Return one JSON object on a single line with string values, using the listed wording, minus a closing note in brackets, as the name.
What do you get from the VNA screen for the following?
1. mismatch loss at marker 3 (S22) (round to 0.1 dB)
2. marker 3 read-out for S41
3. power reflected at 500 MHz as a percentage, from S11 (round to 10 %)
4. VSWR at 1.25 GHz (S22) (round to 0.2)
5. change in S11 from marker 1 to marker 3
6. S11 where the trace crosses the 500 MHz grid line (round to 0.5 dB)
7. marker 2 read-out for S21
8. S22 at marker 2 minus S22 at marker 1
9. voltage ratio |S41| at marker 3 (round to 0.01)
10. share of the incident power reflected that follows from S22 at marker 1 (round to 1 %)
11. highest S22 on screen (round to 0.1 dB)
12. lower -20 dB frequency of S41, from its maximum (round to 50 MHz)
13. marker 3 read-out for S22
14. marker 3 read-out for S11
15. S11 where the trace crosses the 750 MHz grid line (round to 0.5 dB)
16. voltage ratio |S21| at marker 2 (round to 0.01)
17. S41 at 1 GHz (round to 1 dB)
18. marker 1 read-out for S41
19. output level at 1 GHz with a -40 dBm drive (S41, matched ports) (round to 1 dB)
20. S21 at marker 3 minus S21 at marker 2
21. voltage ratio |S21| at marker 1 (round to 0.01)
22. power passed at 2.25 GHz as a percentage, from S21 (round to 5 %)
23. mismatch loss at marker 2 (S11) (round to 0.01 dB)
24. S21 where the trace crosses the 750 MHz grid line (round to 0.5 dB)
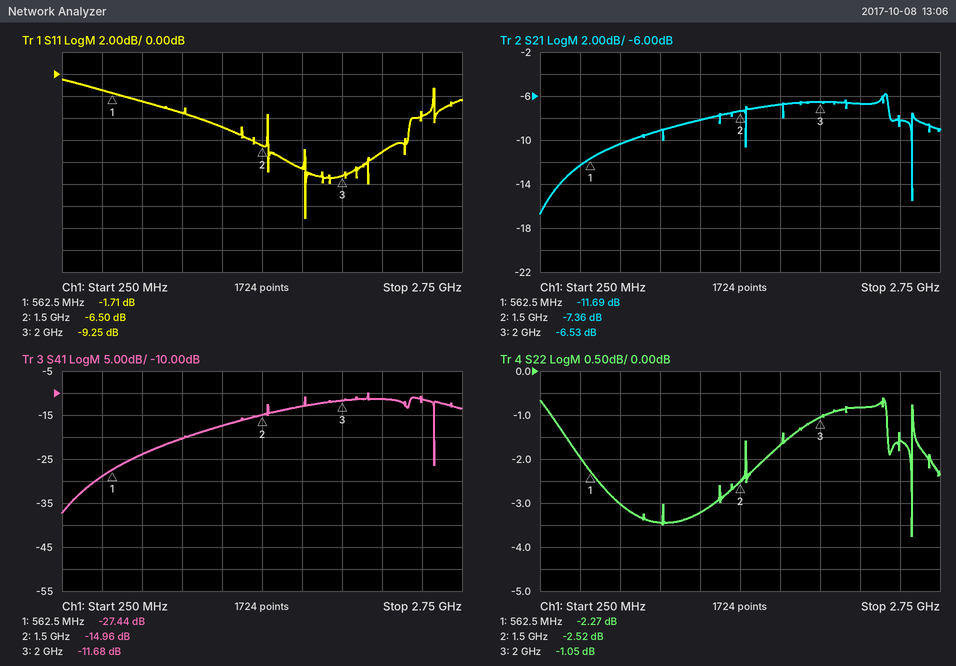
{"mismatch loss at marker 3 (S22)": "6.7 dB", "marker 3 read-out for S41": "-11.68 dB", "power reflected at 500 MHz as a percentage, from S11": "70 %", "VSWR at 1.25 GHz (S22)": "5.4", "change in S11 from marker 1 to marker 3": "-7.54 dB", "S11 where the trace crosses the 500 MHz grid line": "-1.5 dB", "marker 2 read-out for S21": "-7.36 dB", "S22 at marker 2 minus S22 at marker 1": "-0.25 dB", "voltage ratio |S41| at marker 3": "0.26", "share of the incident power reflected that follows from S22 at marker 1": "59 %", "highest S22 on screen": "-0.6 dB", "lower -20 dB frequency of S41, from its maximum": "450 MHz", "marker 3 read-out for S22": "-1.05 dB", "marker 3 read-out for S11": "-9.25 dB", "S11 where the trace crosses the 750 MHz grid line": "-2.5 dB", "voltage ratio |S21| at marker 2": "0.43", "S41 at 1 GHz": "-20 dB", "marker 1 read-out for S41": "-27.44 dB", "output level at 1 GHz with a -40 dBm drive (S41, matched ports)": "-60 dBm", "S21 at marker 3 minus S21 at marker 2": "0.83 dB", "voltage ratio |S21| at marker 1": "0.26", "power passed at 2.25 GHz as a percentage, from S21": "20 %", "mismatch loss at marker 2 (S11)": "1.10 dB", "S21 where the trace crosses the 750 MHz grid line": "-10.5 dB"}
